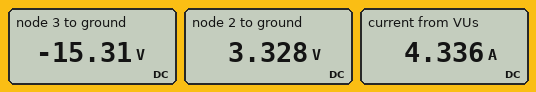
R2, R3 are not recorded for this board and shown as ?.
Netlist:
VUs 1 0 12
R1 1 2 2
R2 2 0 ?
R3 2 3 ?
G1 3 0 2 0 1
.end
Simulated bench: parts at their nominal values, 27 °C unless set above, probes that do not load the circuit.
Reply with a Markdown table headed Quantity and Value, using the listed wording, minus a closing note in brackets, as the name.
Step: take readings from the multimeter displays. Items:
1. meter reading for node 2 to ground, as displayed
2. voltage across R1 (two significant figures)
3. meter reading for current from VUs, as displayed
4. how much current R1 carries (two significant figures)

| Quantity | Value |
|---|---|
| meter reading for node 2 to ground, as displayed | 3.328 V |
| voltage across R1 | 8.7 V |
| meter reading for current from VUs, as displayed | 4.336 A |
| how much current R1 carries | 4.3 A |
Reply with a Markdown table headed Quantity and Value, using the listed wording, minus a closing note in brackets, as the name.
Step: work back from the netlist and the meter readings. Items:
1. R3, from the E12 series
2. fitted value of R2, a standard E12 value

| Quantity | Value |
|---|---|
| R3, from the E12 series | 5.6 Ω |
| fitted value of R2, a standard E12 value | 3.3 Ω |
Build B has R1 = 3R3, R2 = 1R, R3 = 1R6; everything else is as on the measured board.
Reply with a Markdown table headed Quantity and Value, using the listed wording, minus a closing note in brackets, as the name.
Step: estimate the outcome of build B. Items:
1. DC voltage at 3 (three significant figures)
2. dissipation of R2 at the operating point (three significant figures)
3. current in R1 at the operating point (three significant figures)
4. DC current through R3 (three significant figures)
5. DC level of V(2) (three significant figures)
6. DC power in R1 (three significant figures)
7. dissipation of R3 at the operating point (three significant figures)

| Quantity | Value |
|---|---|
| DC voltage at 3 | -947 mV |
| dissipation of R2 at the operating point | 2.49 W |
| current in R1 at the operating point | 3.16 A |
| DC current through R3 | 1.58 A |
| DC level of V(2) | 1.58 V |
| DC power in R1 | 32.9 W |
| dissipation of R3 at the operating point | 3.99 W |
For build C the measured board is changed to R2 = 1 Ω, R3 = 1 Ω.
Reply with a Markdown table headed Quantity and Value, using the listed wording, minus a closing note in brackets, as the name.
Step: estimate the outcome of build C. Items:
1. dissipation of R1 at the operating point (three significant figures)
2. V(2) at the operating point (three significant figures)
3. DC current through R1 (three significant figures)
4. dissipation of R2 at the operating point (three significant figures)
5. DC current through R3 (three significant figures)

| Quantity | Value |
|---|---|
| dissipation of R1 at the operating point | 46.1 W |
| V(2) at the operating point | 2.40 V |
| DC current through R1 | 4.80 A |
| dissipation of R2 at the operating point | 5.76 W |
| DC current through R3 | 2.40 A |
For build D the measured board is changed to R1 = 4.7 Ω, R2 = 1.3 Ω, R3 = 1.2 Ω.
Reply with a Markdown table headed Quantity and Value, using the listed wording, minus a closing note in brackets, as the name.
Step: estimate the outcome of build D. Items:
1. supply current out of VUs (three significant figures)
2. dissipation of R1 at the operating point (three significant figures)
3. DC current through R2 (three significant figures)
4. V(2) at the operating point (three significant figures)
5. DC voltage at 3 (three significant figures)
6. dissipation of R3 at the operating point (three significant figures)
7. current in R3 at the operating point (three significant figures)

| Quantity | Value |
|---|---|
| supply current out of VUs | 2.28 A |
| dissipation of R1 at the operating point | 24.4 W |
| DC current through R2 | 991 mA |
| V(2) at the operating point | 1.29 V |
| DC voltage at 3 | -258 mV |
| dissipation of R3 at the operating point | 1.99 W |
| current in R3 at the operating point | 1.29 A |
